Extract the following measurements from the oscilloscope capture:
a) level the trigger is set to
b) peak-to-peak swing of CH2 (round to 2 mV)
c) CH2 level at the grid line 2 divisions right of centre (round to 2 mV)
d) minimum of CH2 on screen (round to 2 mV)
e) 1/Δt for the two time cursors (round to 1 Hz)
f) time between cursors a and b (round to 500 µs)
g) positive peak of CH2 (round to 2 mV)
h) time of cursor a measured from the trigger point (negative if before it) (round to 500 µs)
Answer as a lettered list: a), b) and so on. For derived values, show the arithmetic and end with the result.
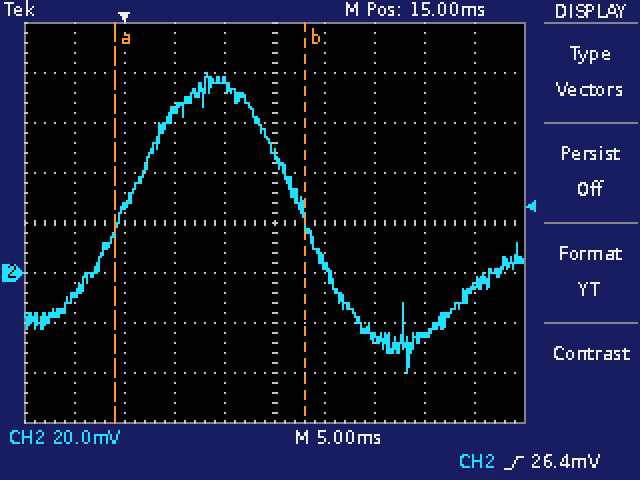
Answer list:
a) 26.4 mV
b) 80 mV − (-40 mV) = 120 mV
c) -26 mV
d) -40 mV
e) 1 / 19.0 ms ≈ 53 Hz
f) 19.0 ms
g) 80 mV
h) -1.0 ms
